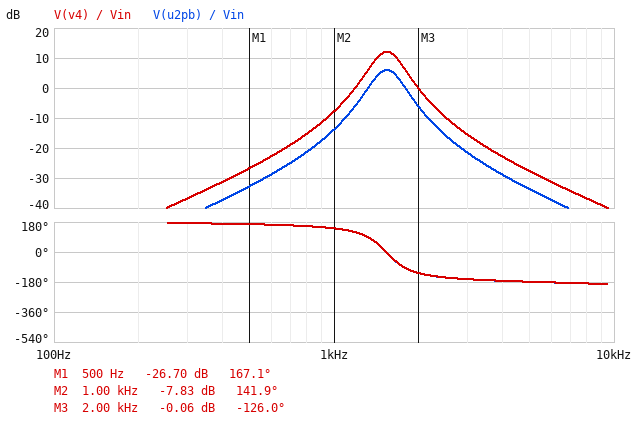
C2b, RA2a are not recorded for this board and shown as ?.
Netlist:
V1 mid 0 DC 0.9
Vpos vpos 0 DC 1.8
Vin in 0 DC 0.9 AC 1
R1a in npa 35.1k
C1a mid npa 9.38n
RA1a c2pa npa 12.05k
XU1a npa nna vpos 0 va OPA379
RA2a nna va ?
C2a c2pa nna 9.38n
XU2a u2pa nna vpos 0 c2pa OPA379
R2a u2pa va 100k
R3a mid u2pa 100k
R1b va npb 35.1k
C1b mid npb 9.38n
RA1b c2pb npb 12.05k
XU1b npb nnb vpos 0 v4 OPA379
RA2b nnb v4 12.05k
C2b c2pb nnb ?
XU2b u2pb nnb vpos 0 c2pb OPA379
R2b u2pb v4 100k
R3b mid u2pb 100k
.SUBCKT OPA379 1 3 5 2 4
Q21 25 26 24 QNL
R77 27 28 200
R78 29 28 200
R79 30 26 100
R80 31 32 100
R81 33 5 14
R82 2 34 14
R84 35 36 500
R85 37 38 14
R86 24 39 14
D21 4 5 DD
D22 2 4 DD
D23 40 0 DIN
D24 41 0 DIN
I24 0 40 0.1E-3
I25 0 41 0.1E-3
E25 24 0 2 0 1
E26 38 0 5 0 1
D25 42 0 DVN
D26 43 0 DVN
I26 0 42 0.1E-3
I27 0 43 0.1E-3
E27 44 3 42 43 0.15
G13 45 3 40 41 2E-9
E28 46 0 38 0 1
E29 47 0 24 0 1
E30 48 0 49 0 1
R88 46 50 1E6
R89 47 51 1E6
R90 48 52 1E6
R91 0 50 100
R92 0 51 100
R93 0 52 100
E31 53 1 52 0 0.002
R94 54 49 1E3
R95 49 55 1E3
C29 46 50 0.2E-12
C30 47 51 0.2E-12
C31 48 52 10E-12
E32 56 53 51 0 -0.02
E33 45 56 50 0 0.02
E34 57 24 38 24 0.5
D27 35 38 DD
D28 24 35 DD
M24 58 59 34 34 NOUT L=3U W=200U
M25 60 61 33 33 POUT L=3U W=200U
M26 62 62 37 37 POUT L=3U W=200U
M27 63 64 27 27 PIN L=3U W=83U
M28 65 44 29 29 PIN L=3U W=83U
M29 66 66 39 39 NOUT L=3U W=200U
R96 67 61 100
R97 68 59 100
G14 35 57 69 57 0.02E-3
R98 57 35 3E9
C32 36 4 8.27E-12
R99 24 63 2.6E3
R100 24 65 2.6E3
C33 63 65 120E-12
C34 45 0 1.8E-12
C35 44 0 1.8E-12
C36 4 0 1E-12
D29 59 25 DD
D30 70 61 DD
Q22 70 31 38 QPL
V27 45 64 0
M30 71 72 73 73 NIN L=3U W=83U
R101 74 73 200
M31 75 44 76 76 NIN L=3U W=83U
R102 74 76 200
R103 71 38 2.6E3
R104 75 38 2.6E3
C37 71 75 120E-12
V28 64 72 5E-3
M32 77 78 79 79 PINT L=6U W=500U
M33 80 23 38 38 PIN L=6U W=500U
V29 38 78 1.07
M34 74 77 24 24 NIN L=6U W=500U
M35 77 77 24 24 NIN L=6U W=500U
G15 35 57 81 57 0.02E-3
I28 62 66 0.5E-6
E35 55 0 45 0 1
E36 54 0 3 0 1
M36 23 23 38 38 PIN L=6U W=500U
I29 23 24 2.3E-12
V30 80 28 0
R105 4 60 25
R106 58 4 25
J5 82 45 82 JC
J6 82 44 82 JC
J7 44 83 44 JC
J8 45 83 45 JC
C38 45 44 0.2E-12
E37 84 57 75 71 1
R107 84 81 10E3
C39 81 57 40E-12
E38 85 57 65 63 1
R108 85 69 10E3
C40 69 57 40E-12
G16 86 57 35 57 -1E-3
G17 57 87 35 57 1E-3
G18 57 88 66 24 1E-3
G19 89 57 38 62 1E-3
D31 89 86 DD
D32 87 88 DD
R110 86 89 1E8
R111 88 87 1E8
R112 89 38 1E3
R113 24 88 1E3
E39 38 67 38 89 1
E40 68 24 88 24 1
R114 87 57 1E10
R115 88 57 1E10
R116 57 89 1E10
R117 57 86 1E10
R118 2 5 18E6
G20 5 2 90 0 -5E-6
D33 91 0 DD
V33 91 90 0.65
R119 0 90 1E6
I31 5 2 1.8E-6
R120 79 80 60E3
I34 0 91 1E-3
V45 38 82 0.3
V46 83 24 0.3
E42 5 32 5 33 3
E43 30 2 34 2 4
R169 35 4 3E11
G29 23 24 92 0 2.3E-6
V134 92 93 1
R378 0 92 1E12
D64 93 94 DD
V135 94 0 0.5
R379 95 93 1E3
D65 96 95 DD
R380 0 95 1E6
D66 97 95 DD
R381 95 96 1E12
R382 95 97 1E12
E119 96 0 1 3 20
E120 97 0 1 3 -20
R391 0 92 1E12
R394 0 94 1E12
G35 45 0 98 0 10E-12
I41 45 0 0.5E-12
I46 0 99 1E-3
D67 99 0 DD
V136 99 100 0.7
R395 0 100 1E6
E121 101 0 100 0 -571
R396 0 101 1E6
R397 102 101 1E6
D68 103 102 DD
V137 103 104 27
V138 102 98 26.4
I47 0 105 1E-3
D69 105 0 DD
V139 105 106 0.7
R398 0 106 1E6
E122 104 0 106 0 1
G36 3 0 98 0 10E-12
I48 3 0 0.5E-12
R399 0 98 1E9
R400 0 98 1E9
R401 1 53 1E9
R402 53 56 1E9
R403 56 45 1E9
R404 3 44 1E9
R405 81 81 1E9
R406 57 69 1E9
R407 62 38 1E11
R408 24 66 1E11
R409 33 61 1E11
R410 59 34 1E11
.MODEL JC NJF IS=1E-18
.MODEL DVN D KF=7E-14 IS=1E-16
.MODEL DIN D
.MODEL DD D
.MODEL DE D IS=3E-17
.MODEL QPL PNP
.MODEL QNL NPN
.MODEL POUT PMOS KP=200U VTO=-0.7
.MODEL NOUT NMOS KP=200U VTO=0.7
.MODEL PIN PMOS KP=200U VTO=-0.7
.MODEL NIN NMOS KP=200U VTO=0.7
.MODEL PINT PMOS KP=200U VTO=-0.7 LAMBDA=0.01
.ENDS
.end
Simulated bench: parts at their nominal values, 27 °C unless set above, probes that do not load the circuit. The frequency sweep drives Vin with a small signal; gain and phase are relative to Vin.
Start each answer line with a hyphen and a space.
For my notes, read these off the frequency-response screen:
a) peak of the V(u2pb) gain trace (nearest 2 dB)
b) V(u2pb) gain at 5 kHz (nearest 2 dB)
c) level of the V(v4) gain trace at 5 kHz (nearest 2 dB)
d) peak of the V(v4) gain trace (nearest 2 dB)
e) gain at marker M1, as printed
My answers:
- 6 dB
- -34 dB
- -28 dB
- 12 dB
- -26.70 dB
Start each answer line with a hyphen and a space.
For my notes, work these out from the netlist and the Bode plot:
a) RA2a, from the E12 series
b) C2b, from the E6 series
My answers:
- 10 kΩ
- 6.8 nF
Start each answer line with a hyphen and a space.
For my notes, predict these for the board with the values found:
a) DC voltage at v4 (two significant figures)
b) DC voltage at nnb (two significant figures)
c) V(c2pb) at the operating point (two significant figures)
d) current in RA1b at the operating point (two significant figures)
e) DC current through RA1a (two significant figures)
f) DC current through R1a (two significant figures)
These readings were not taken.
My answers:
- 890 mV
- 890 mV
- 900 mV
- 140 nA
- 140 nA
- 140 nA
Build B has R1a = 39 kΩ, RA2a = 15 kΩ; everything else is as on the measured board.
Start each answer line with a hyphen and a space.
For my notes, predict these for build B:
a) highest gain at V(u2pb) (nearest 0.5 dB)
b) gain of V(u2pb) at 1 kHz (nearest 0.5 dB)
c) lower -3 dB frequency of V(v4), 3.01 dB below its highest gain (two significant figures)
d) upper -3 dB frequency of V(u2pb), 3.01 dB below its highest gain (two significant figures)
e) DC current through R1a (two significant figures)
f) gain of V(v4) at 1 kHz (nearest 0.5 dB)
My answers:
- 1.5 dB
- -8.5 dB
- 1.2 kHz
- 1.7 kHz
- 130 nA
- -2.5 dB
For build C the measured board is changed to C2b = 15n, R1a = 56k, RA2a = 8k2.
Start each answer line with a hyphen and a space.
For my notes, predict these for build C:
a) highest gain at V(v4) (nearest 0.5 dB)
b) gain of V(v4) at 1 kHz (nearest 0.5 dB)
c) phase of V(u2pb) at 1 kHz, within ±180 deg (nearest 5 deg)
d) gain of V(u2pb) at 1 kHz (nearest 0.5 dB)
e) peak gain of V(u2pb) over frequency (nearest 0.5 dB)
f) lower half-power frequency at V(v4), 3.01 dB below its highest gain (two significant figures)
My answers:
- 6.5 dB
- -4.0 dB
- 100 deg
- -10.0 dB
- 0.5 dB
- 1.5 kHz
